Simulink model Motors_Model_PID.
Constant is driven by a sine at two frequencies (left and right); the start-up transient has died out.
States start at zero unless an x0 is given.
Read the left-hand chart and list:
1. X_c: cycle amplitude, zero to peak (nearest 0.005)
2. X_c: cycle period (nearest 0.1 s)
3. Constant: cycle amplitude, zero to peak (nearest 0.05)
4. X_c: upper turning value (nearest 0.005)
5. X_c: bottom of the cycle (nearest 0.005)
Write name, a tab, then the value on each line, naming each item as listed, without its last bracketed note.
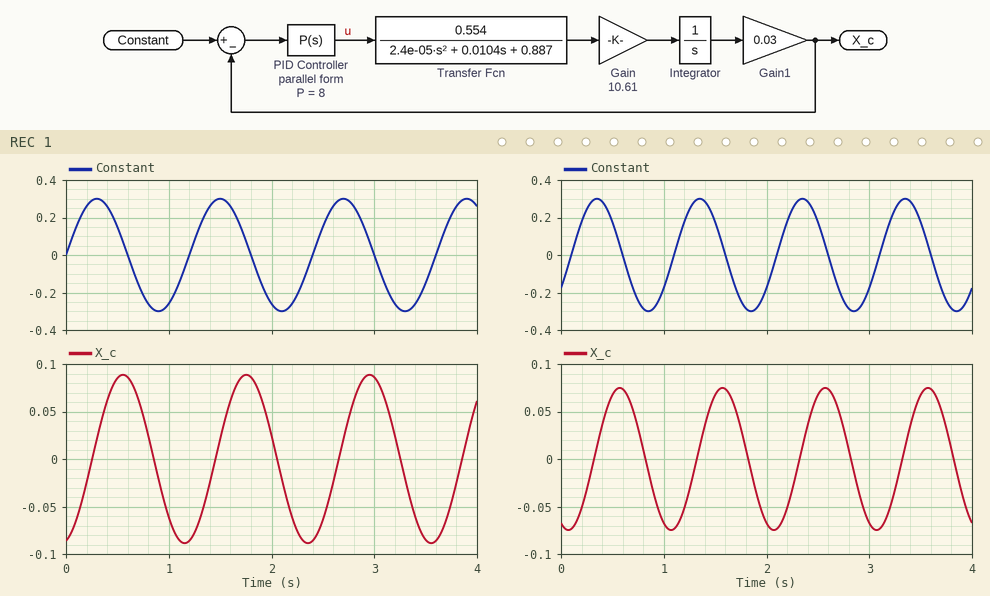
X_c: cycle amplitude, zero to peak	0.090
X_c: cycle period	1.2 s
Constant: cycle amplitude, zero to peak	0.30
X_c: upper turning value	0.090
X_c: bottom of the cycle	-0.090
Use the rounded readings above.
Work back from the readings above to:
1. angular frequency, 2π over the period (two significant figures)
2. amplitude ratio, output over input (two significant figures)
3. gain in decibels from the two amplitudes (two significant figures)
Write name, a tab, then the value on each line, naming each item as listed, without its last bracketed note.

angular frequency, 2π over the period	5.2 rad/s
amplitude ratio, output over input	0.30
gain in decibels from the two amplitudes	-10 dB
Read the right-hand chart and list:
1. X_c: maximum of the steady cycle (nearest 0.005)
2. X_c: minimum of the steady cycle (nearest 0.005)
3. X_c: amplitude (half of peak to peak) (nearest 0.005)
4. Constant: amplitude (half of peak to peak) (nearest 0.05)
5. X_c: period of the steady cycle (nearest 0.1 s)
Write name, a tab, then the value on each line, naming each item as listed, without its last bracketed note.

X_c: maximum of the steady cycle	0.075
X_c: minimum of the steady cycle	-0.075
X_c: amplitude (half of peak to peak)	0.075
Constant: amplitude (half of peak to peak)	0.30
X_c: period of the steady cycle	1.0 s
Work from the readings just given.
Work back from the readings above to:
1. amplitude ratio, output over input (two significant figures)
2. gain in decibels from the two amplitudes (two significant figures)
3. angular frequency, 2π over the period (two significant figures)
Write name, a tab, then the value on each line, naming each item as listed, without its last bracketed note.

amplitude ratio, output over input	0.25
gain in decibels from the two amplitudes	-12 dB
angular frequency, 2π over the period	6.3 rad/s
